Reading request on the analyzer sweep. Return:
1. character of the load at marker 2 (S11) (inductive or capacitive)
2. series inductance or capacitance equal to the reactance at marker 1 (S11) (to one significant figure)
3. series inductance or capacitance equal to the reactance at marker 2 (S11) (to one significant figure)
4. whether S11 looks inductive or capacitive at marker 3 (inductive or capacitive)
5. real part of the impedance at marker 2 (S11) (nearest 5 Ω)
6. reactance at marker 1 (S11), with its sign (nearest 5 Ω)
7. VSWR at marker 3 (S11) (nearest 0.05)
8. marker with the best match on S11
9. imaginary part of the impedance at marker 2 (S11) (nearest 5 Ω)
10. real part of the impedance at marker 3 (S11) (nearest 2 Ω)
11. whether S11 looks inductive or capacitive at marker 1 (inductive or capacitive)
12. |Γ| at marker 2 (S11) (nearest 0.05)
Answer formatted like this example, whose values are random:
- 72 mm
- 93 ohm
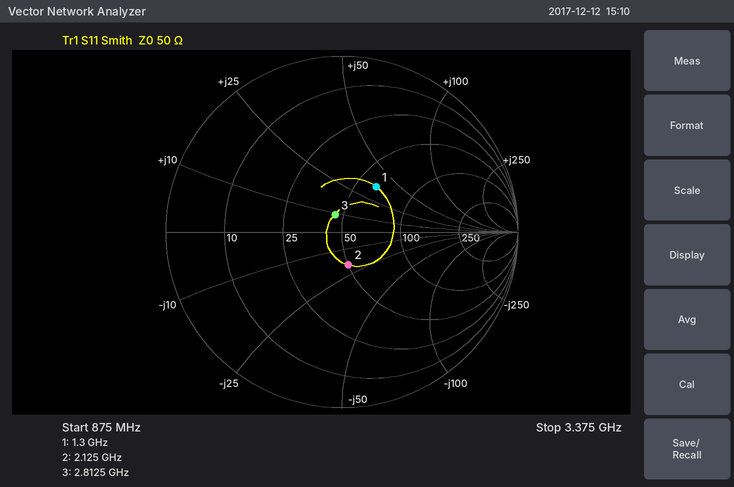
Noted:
- capacitive
- 4 nH
- 4 pF
- inductive
- 50 Ω
- +35 Ω
- 1.25
- marker 3
- -20 Ω
- 46 Ω
- inductive
- 0.20
